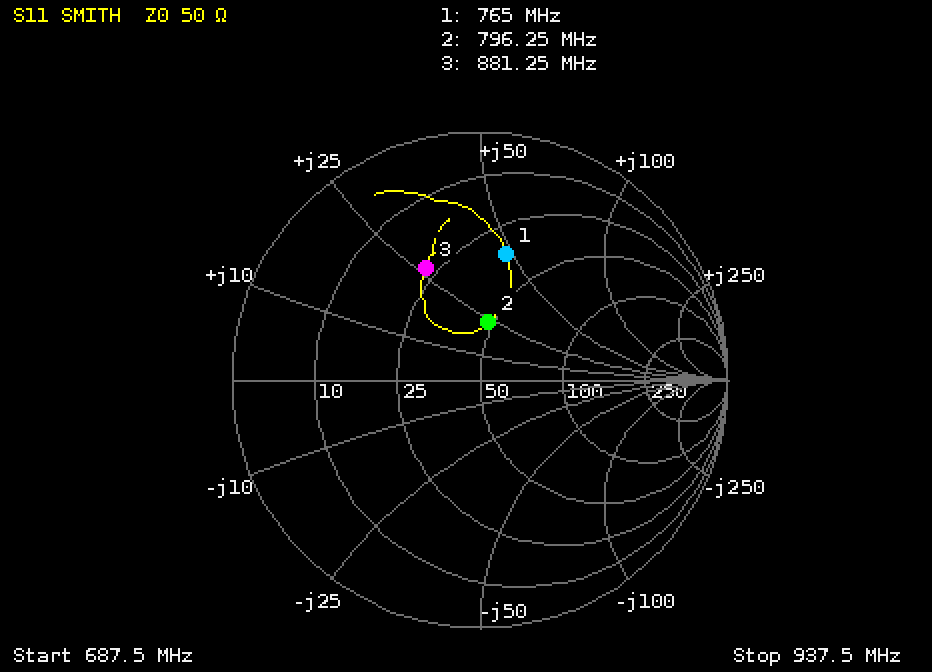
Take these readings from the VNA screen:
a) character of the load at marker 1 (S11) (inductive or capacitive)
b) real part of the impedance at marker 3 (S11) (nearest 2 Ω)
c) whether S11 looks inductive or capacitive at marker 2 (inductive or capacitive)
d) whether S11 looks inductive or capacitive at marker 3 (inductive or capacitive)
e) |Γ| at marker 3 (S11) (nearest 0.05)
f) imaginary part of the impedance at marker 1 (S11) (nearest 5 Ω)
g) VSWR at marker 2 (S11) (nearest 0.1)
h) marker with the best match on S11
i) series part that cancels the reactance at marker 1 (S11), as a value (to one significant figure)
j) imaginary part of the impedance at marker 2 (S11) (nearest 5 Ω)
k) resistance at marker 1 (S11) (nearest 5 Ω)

inductive
22 Ω
inductive
inductive
0.50
+50 Ω
1.6
marker 2
4 pF
+25 Ω
35 Ω
